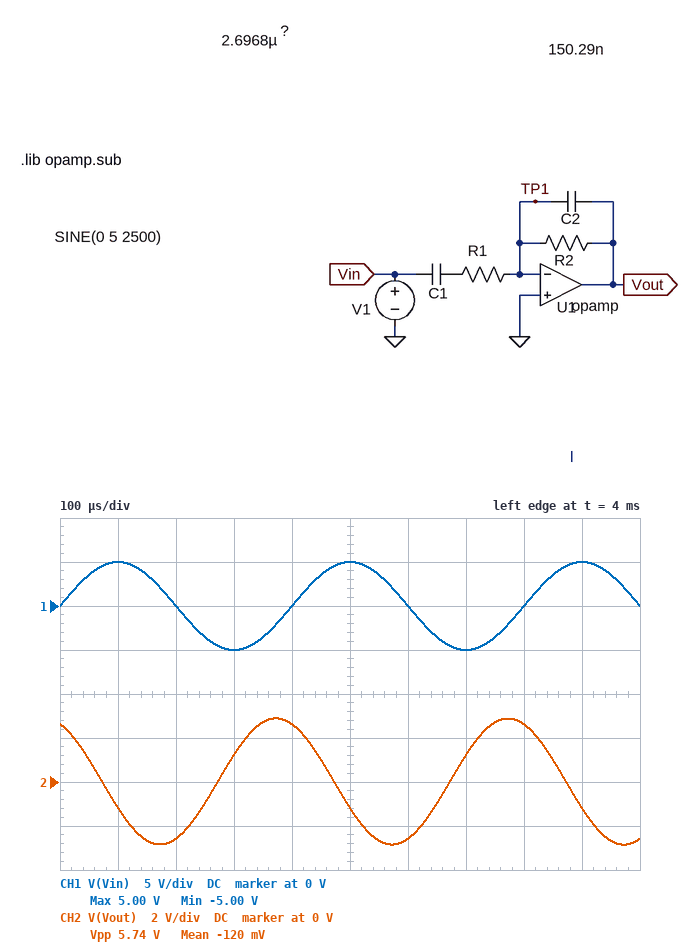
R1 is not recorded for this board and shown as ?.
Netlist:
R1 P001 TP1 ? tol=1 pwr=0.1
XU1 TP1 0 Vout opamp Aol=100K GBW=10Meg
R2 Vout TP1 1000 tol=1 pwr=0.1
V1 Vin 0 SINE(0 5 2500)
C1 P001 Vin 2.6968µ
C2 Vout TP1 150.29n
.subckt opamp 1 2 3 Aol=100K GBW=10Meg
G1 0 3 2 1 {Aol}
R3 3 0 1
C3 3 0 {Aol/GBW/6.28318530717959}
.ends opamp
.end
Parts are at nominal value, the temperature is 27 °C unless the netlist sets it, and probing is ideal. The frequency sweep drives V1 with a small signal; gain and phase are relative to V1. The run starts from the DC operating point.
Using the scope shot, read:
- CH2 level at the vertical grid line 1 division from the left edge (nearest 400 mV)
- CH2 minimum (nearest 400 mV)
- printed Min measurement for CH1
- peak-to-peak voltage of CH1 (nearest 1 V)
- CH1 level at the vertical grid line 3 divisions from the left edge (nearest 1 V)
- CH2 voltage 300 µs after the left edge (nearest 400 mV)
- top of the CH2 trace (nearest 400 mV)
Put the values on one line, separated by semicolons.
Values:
-1.2 V; -2.8 V; -5.00 V; 10 V; -5 V; 1.2 V; 2.8 V
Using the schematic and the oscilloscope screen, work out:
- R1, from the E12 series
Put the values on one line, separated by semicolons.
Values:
680 Ω
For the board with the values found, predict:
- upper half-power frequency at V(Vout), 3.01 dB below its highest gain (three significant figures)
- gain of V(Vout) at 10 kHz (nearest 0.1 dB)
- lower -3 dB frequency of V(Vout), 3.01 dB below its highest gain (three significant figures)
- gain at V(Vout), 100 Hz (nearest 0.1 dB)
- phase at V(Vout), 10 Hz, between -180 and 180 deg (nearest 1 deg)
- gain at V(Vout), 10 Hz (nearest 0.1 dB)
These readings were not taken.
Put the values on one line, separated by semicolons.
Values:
1.22 kHz; -16.2 dB; 75.3 Hz; 0.9 dB; -97 deg; -15.5 dB
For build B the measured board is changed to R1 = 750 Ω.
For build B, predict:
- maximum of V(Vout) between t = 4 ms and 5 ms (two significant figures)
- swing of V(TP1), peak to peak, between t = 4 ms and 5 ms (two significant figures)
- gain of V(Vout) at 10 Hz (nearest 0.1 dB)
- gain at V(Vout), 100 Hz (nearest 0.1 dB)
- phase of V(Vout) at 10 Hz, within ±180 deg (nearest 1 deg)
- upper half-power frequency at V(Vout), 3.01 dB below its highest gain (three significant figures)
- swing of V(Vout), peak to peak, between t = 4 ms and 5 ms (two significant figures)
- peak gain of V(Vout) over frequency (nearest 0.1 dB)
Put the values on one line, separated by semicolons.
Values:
2.6 V; 1.3 mV; -15.5 dB; 0.4 dB; -98 deg; 1.21 kHz; 5.2 V; 1.9 dB
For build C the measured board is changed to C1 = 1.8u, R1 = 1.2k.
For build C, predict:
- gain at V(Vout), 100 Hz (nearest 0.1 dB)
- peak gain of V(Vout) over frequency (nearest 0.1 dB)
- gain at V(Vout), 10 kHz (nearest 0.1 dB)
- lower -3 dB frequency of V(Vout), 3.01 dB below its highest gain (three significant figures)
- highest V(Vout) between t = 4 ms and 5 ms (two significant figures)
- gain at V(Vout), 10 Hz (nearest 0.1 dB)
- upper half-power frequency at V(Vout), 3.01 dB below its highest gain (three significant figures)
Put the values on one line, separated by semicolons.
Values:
-3.5 dB; -2.2 dB; -21.1 dB; 65.1 Hz; 1.6 V; -19.0 dB; 1.20 kHz
